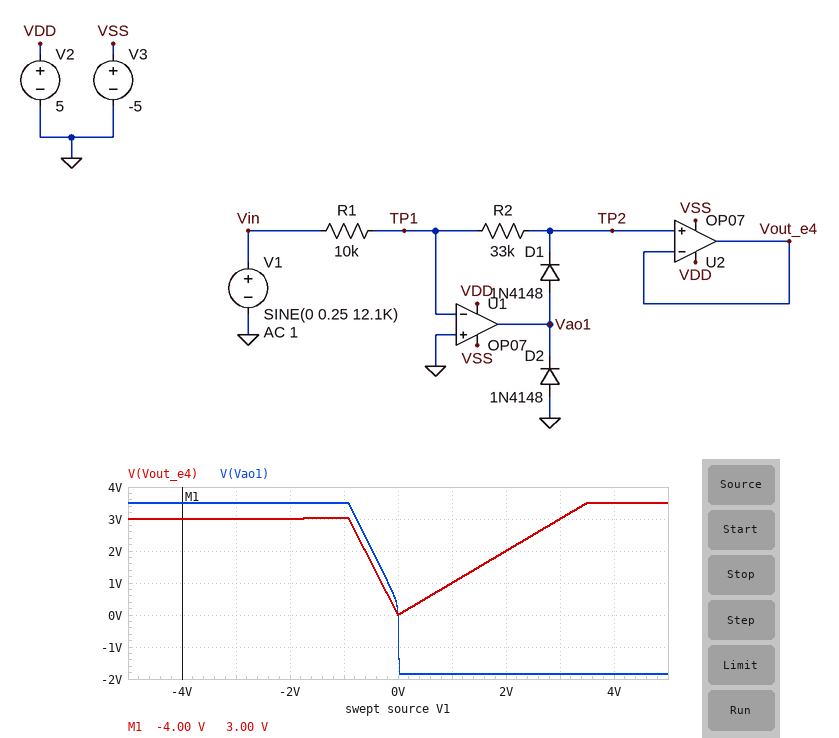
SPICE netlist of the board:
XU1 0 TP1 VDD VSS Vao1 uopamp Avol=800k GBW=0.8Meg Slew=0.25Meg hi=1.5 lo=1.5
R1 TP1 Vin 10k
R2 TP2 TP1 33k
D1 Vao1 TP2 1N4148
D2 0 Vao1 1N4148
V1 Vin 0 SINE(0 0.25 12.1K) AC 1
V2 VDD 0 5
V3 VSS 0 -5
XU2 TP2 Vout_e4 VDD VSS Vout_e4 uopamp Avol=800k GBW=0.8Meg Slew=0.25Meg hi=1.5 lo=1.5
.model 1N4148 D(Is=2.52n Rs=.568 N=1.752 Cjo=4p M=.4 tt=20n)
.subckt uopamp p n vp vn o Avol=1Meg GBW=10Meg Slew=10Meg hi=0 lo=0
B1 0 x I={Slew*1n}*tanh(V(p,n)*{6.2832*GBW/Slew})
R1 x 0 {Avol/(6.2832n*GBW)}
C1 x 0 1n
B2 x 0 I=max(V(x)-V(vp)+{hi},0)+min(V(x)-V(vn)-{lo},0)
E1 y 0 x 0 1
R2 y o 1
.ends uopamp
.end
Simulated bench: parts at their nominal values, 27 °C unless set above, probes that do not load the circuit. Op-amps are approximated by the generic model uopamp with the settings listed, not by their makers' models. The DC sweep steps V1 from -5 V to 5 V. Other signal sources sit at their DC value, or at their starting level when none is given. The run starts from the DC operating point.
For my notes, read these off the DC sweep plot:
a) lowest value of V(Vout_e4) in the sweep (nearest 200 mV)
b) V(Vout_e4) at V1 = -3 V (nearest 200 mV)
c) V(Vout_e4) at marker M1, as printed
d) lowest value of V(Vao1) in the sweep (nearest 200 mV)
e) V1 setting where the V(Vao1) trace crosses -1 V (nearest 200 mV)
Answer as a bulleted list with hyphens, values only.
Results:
- 0 V
- 3.0 V
- 3.00 V
- -1.8 V
- 0 V
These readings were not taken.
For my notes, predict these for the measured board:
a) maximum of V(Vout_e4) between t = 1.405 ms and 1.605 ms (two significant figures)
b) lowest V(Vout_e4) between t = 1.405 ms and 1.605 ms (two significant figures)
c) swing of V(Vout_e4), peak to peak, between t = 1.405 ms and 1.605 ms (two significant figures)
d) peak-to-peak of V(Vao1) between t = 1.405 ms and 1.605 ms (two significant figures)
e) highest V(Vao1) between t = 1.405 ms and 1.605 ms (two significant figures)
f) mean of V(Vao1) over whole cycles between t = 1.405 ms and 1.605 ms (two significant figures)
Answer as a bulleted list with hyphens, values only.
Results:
- 810 mV
- -190 mV
- 990 mV
- 3.1 V
- 1.2 V
- -680 mV
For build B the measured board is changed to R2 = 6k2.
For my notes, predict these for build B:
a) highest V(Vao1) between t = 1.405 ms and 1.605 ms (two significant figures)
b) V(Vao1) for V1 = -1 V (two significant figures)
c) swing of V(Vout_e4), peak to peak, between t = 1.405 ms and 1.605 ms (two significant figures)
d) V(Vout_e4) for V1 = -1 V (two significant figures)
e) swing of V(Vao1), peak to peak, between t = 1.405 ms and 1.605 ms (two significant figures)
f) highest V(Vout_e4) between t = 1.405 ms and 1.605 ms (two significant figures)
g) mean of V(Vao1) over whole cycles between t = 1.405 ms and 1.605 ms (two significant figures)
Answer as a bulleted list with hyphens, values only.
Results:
- 570 mV
- 1.1 V
- 460 mV
- 620 mV
- 2.4 V
- 250 mV
- -810 mV
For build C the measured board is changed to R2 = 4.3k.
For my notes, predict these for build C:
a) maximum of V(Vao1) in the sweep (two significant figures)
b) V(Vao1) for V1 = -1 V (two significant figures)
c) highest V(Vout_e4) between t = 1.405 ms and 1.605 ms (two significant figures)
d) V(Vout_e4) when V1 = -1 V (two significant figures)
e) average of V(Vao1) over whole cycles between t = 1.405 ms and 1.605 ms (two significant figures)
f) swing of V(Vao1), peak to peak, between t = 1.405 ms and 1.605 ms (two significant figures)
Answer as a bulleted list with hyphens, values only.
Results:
- 2.7 V
- 910 mV
- 250 mV
- 430 mV
- -820 mV
- 2.4 V
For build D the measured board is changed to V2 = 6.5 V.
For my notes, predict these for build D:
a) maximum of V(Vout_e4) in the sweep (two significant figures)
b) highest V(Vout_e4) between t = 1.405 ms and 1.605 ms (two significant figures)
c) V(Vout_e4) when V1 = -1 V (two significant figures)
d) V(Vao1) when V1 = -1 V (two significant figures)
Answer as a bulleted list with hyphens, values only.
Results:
- 5.0 V
- 810 mV
- 3.3 V
- 3.8 V
